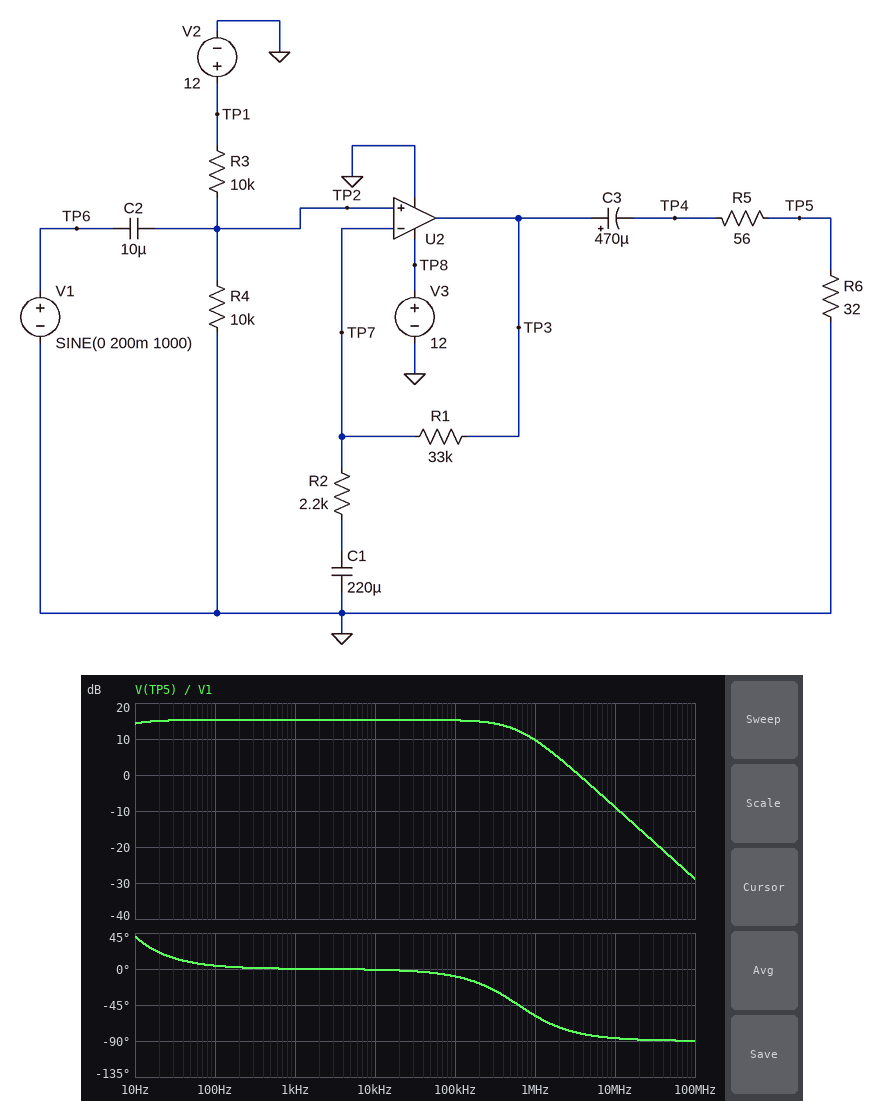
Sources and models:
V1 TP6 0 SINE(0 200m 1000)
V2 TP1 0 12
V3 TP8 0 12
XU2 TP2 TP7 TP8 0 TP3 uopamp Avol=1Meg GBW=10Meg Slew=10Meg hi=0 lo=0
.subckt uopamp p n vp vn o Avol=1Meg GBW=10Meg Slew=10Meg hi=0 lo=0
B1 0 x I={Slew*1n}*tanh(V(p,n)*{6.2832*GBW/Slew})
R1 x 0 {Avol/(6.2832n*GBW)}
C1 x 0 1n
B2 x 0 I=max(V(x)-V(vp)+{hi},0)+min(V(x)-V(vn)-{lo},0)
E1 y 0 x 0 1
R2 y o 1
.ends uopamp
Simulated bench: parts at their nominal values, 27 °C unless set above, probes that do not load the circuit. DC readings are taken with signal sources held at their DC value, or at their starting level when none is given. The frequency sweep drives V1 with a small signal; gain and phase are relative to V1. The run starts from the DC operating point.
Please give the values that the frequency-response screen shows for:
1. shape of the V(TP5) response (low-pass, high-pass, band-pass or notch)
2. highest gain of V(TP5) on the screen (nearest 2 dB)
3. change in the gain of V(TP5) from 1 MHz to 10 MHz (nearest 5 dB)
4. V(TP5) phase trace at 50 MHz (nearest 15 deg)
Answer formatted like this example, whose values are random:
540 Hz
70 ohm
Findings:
low-pass
16 dB
-20 dB
-90 deg
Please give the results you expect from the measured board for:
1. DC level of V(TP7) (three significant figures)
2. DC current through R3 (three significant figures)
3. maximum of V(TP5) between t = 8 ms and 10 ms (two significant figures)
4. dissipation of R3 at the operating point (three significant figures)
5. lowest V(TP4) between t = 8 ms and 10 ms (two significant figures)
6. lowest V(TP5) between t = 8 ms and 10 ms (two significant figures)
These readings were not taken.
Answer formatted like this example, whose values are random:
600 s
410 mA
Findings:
6.00 V
600 µA
1.2 V
3.60 mW
-3.2 V
-1.2 V
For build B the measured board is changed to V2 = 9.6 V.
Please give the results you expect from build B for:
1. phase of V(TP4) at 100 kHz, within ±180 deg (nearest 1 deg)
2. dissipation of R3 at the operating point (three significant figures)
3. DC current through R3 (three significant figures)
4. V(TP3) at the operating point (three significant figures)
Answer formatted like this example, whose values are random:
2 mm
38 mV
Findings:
-9 deg
2.30 mW
480 µA
4.80 V
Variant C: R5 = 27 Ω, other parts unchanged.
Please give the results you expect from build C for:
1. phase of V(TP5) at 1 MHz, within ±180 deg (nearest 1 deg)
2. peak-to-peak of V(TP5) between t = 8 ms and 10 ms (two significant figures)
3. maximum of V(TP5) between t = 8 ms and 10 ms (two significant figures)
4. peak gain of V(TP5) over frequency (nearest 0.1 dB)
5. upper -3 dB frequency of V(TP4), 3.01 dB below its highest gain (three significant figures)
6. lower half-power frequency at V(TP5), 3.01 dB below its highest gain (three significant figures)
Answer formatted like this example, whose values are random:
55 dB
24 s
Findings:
-58 deg
3.5 V
1.7 V
18.8 dB
615 kHz
7.07 Hz
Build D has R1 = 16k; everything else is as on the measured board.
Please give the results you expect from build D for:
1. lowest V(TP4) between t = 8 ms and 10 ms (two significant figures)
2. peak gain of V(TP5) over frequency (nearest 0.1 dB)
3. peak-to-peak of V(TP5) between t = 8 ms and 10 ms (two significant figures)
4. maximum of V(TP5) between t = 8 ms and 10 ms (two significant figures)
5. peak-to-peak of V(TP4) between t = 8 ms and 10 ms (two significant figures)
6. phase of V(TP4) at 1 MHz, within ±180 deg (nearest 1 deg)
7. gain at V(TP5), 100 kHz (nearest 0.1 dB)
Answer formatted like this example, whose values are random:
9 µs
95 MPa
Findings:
-1.7 V
9.6 dB
1.2 V
600 mV
3.3 V
-40 deg
9.5 dB
